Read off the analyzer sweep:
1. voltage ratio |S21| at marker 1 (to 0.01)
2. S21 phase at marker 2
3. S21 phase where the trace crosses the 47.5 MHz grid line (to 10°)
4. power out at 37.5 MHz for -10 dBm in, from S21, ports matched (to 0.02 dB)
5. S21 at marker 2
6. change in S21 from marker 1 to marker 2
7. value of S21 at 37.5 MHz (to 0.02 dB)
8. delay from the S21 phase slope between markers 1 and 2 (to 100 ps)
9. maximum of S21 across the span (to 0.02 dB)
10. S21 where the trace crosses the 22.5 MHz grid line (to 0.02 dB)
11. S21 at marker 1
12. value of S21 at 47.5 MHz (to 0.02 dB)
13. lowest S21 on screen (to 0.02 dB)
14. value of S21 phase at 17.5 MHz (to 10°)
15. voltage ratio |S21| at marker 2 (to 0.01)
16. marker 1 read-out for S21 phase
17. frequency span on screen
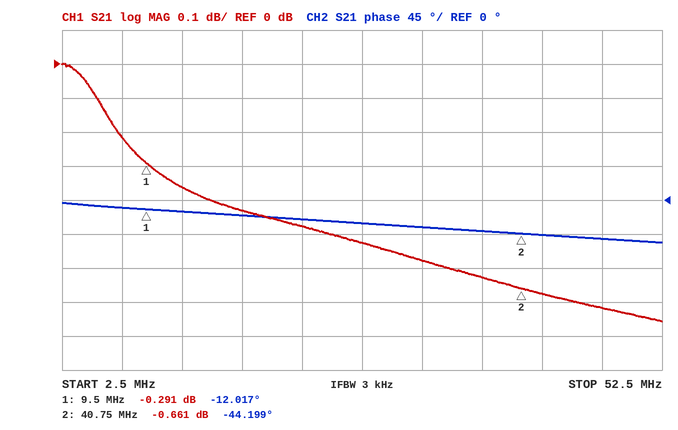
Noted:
0.97
-44.199°
-50°
-10.62 dBm
-0.661 dB
-0.370 dB
-0.62 dB
2.9 ns
0.00 dB
-0.48 dB
-0.291 dB
-0.72 dB
-0.76 dB
-20°
0.93
-12.017°
50 MHz
